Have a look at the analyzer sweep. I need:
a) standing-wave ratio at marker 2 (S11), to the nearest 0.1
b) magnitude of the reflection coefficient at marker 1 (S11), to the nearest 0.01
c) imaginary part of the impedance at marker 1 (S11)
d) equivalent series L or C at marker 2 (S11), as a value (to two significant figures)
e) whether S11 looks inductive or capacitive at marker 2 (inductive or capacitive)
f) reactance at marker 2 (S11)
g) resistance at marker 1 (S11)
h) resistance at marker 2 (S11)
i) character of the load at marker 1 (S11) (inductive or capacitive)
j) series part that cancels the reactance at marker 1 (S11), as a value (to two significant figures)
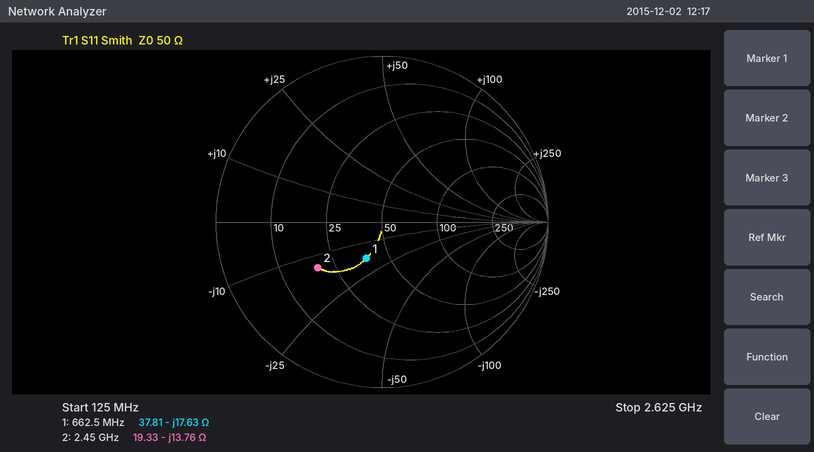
2.8
0.24
-17.63 Ω
4.7 pF
capacitive
-13.76 Ω
37.81 Ω
19.33 Ω
capacitive
4.2 nH
